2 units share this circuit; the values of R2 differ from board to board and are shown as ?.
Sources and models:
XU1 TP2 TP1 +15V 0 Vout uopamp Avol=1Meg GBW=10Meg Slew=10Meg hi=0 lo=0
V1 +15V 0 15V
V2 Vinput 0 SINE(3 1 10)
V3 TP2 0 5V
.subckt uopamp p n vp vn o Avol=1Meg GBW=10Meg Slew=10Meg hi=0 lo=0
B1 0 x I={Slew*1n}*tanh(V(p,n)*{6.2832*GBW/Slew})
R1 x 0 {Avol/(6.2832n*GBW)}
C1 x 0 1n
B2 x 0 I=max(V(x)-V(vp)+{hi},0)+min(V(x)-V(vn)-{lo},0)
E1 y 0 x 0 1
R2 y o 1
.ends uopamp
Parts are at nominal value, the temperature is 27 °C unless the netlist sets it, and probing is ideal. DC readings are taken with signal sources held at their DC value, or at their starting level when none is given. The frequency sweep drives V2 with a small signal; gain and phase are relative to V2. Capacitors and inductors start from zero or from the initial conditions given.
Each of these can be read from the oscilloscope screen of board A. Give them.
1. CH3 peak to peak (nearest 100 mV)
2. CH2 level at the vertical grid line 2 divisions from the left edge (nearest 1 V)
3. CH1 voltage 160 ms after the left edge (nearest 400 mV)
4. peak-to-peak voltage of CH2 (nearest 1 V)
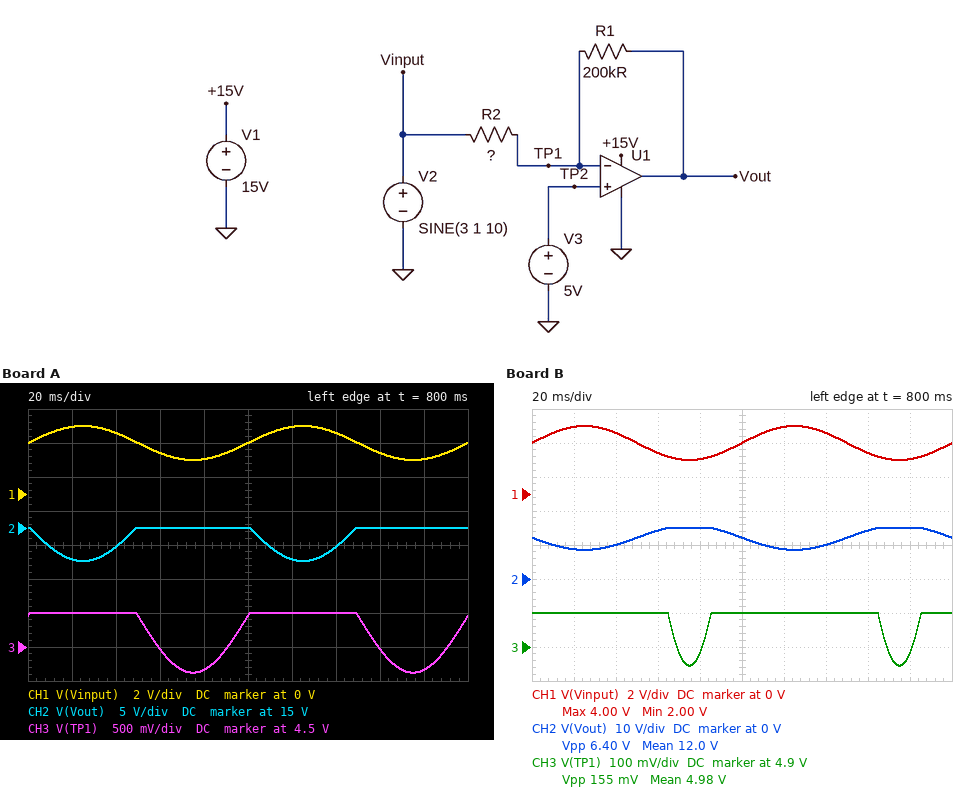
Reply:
900 mV
12 V
2.4 V
5 V
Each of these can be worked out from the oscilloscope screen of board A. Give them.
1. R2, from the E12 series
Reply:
39 kΩ
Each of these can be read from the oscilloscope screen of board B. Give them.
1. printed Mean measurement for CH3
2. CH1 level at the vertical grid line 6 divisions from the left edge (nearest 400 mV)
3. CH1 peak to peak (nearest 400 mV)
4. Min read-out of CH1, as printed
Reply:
4.98 V
4.0 V
2.0 V
2.00 V
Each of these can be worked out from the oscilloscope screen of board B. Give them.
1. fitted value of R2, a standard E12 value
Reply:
56 kΩ
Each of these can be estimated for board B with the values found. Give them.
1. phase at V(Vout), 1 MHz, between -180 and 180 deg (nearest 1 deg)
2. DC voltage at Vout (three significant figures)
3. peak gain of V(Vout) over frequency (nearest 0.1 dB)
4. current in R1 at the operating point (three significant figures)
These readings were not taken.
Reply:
155 deg
12.1 V
11.1 dB
35.7 µA
